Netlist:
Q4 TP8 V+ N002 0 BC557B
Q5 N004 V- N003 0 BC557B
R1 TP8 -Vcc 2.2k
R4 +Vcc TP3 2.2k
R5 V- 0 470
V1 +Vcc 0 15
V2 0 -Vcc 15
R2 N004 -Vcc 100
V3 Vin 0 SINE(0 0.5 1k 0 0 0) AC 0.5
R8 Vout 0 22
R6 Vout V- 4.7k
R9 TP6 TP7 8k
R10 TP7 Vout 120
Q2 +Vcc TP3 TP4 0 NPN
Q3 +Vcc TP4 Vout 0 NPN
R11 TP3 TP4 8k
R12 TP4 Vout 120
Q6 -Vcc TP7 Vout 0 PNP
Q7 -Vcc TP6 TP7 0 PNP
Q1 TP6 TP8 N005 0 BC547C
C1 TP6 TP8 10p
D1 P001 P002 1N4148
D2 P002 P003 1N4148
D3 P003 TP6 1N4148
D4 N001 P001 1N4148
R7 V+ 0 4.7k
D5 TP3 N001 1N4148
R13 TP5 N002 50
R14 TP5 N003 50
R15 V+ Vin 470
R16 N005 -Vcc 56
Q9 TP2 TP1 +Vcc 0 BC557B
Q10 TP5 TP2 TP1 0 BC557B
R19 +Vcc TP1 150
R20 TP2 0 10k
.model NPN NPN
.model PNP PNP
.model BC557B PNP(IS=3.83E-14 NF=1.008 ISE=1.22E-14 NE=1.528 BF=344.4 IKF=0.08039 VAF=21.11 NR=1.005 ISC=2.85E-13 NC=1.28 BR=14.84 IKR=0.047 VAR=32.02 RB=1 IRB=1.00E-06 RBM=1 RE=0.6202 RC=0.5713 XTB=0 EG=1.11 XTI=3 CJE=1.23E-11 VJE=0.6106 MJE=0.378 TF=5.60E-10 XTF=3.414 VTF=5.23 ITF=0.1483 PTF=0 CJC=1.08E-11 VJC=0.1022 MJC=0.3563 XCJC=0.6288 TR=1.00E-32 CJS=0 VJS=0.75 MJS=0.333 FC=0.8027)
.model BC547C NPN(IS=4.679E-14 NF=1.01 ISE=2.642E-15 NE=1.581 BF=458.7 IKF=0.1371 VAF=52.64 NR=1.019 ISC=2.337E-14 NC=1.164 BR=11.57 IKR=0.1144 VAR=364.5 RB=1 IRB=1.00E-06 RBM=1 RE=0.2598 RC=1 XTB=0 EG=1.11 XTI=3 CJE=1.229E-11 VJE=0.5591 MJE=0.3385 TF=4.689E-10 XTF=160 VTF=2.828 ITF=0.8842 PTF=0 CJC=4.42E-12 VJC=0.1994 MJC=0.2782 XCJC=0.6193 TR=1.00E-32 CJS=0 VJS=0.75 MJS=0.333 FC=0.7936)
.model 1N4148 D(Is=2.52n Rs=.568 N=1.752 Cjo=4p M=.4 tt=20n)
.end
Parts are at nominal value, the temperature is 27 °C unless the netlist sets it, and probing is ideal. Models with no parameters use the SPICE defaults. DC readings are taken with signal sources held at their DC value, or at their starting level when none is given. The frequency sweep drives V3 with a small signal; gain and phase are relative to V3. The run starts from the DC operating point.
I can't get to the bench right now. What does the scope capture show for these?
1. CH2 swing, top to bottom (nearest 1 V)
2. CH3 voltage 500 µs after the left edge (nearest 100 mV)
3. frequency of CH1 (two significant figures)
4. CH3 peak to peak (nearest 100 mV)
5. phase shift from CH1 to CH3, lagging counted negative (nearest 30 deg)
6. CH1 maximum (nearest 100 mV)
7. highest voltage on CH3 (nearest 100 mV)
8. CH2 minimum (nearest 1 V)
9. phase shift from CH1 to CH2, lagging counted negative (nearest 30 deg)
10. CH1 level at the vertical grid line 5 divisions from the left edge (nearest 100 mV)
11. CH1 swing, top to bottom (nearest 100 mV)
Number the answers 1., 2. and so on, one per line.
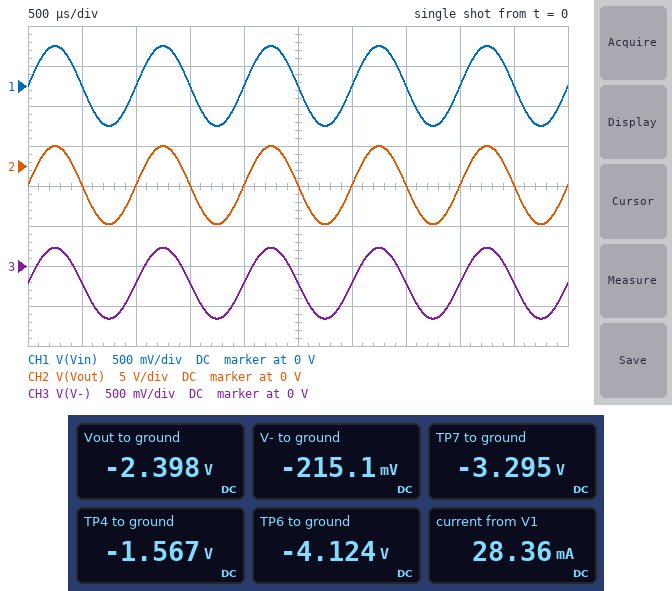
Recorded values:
1. 10 V
2. -200 mV
3. 1.0 kHz
4. 900 mV
5. 0 deg
6. 500 mV
7. 200 mV
8. -7 V
9. 0 deg
10. 0 V
11. 1.0 V
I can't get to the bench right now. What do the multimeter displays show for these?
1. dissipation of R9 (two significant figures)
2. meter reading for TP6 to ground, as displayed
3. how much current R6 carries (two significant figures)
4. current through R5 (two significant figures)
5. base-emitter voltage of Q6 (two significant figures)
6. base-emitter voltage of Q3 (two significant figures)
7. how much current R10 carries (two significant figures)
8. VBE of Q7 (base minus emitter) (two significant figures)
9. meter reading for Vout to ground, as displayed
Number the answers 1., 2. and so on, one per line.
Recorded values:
1. 86 µW
2. -4.124 V
3. 460 µA
4. 460 µA
5. -900 mV
6. 830 mV
7. 7.5 mA
8. -830 mV
9. -2.398 V
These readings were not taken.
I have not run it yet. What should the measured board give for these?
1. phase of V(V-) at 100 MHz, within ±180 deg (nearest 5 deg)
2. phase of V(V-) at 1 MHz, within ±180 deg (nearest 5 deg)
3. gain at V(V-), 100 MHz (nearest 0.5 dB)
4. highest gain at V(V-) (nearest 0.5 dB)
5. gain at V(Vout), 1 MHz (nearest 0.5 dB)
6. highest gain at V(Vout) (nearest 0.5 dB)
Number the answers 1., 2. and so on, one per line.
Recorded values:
1. -20 deg
2. -10 deg
3. -10.5 dB
4. -1.0 dB
5. 20.0 dB
6. 20.0 dB
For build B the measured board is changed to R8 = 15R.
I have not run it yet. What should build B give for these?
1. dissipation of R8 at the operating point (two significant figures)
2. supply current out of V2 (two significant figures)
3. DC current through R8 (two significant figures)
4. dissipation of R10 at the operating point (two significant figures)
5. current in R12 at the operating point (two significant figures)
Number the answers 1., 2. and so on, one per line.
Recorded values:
1. 380 mW
2. 180 mA
3. 160 mA
4. 6.8 mW
5. 6.8 mA
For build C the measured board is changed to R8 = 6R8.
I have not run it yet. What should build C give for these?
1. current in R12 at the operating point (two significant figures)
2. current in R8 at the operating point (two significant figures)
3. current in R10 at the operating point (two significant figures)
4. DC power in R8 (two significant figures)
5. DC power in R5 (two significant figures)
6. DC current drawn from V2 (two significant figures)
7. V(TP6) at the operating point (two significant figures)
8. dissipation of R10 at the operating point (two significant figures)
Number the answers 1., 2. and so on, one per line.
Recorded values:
1. 6.6 mA
2. 350 mA
3. 7.7 mA
4. 840 mW
5. 98 µW
6. 370 mA
7. -4.2 V
8. 7.1 mW
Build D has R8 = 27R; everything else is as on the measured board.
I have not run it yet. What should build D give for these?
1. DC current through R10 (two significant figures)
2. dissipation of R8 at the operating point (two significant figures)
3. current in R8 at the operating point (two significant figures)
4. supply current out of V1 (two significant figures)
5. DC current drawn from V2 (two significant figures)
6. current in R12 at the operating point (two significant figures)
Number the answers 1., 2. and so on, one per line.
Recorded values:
1. 7.4 mA
2. 210 mW
3. 89 mA
4. 30 mA
5. 120 mA
6. 7.0 mA
